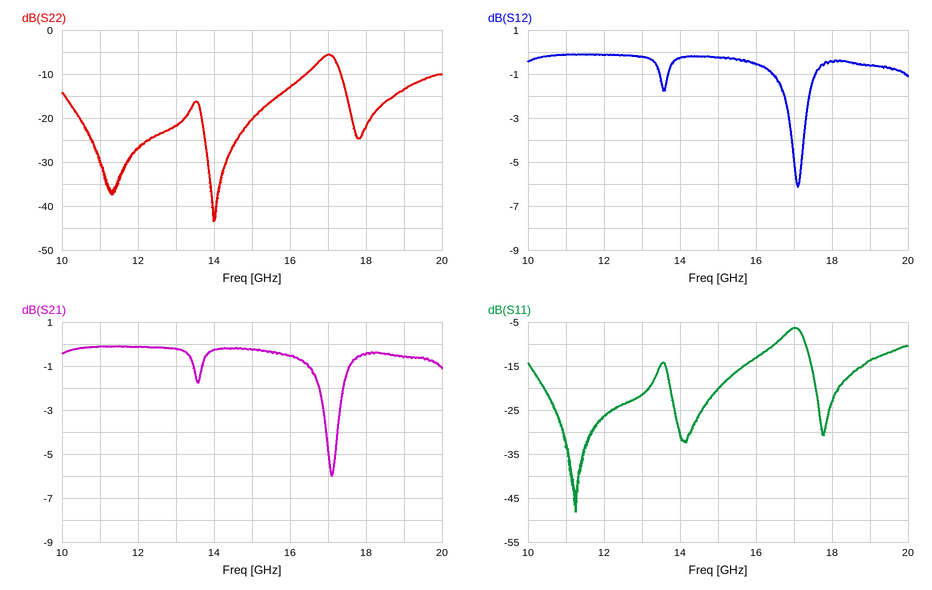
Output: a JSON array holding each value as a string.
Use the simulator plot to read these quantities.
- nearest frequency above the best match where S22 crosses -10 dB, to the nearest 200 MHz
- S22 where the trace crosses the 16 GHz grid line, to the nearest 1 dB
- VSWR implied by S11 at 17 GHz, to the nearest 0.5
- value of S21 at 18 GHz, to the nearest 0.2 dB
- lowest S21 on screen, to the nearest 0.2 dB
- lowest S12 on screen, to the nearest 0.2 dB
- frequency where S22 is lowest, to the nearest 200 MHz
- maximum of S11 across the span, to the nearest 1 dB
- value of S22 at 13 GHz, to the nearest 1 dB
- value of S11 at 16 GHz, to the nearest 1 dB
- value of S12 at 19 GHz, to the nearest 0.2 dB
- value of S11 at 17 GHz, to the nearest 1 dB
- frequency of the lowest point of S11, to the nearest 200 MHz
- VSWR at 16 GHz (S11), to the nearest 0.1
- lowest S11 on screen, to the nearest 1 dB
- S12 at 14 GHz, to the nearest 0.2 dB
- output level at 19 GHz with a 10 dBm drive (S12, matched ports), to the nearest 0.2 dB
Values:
["16.4 GHz", "-13 dB", "3.0", "-0.4 dB", "-6.0 dB", "-6.2 dB", "14.0 GHz", "-6 dB", "-22 dB", "-13 dB", "-0.6 dB", "-6 dB", "11.2 GHz", "1.6", "-48 dB", "-0.2 dB", "9.4 dBm"]
